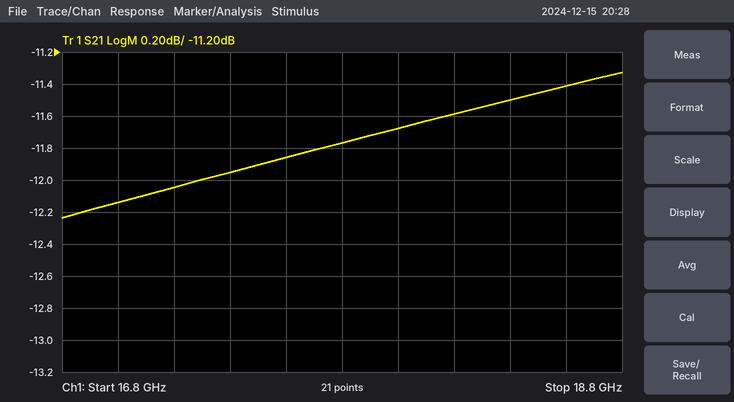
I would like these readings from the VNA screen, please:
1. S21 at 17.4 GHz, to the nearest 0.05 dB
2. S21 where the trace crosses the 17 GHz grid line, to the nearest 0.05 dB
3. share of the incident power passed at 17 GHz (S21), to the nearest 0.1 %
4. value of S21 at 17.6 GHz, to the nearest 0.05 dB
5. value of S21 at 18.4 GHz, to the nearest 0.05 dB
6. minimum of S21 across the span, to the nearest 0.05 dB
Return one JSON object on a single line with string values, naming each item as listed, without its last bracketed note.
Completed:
{"S21 at 17.4 GHz, to the nearest 0.05 dB": "-11.95 dB", "S21 where the trace crosses the 17 GHz grid line, to the nearest 0.05 dB": "-12.15 dB", "share of the incident power passed at 17 GHz (S21), to the nearest 0.1 %": "6.1 %", "value of S21 at 17.6 GHz, to the nearest 0.05 dB": "-11.85 dB", "value of S21 at 18.4 GHz, to the nearest 0.05 dB": "-11.50 dB", "minimum of S21 across the span, to the nearest 0.05 dB": "-12.25 dB"}
